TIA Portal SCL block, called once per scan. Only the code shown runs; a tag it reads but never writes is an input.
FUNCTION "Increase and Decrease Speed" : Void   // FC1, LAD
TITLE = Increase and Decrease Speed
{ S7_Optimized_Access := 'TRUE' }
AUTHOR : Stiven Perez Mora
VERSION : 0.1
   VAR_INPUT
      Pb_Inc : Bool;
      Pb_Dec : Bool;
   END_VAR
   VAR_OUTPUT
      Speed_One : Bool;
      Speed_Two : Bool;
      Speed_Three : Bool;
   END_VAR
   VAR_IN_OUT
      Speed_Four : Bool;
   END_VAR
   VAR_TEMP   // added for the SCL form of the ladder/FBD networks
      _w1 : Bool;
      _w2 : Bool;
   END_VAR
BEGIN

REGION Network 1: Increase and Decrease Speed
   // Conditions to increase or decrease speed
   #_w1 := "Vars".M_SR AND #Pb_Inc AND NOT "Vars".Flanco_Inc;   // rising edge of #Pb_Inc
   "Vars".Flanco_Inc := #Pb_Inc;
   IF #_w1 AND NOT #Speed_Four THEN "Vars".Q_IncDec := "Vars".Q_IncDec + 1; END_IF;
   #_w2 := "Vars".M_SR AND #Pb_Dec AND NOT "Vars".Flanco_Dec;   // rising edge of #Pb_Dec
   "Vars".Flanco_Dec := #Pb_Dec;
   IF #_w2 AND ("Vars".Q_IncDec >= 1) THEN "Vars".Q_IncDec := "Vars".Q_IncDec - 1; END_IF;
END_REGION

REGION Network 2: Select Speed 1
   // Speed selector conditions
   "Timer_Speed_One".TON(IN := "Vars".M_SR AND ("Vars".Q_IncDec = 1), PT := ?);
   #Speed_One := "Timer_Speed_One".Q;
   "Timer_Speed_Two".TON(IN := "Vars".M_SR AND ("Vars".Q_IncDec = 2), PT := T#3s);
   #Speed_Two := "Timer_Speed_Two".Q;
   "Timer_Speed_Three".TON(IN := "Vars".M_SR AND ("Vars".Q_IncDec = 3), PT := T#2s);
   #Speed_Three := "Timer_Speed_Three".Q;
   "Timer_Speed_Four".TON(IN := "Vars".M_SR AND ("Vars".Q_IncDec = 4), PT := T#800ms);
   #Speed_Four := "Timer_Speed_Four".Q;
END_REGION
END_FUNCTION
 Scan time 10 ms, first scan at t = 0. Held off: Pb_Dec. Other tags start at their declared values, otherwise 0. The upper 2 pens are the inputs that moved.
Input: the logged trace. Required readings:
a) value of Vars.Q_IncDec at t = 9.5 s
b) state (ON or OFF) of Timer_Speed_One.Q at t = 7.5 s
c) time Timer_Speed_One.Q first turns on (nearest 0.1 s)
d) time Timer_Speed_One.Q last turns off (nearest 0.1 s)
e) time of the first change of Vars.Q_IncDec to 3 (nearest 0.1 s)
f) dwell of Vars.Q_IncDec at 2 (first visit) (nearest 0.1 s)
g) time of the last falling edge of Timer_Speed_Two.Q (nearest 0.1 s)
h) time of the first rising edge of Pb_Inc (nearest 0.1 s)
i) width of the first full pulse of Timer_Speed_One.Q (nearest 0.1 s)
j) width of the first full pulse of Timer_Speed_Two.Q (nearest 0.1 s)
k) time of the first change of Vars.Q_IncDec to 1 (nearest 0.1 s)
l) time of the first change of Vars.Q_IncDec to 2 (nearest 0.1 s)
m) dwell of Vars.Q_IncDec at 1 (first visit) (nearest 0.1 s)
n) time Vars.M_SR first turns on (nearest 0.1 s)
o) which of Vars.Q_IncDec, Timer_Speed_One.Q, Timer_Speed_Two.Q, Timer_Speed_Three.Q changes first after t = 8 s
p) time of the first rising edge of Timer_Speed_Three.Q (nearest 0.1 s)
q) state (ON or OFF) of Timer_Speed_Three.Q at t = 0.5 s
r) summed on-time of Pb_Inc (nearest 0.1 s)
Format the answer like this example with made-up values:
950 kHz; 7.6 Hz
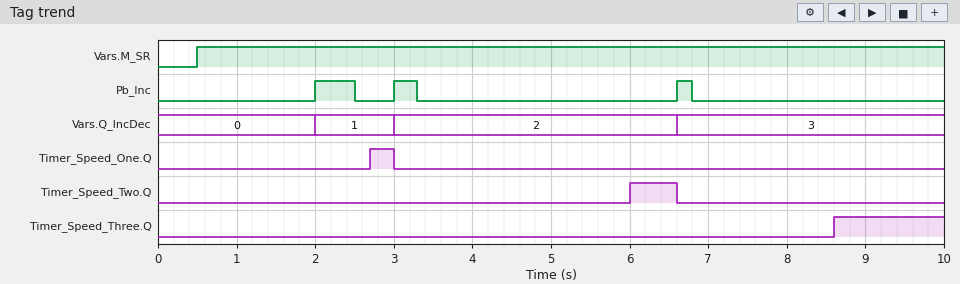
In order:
3; OFF; 2.7 s; 3.0 s; 6.6 s; 3.6 s; 6.6 s; 2.0 s; 0.3 s; 0.6 s; 2.0 s; 3.0 s; 1.0 s; 0.5 s; Timer_Speed_Three.Q; 8.6 s; OFF; 1.0 s
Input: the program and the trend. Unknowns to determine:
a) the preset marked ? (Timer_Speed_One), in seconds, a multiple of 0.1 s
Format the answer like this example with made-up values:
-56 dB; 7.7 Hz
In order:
0.7 s
